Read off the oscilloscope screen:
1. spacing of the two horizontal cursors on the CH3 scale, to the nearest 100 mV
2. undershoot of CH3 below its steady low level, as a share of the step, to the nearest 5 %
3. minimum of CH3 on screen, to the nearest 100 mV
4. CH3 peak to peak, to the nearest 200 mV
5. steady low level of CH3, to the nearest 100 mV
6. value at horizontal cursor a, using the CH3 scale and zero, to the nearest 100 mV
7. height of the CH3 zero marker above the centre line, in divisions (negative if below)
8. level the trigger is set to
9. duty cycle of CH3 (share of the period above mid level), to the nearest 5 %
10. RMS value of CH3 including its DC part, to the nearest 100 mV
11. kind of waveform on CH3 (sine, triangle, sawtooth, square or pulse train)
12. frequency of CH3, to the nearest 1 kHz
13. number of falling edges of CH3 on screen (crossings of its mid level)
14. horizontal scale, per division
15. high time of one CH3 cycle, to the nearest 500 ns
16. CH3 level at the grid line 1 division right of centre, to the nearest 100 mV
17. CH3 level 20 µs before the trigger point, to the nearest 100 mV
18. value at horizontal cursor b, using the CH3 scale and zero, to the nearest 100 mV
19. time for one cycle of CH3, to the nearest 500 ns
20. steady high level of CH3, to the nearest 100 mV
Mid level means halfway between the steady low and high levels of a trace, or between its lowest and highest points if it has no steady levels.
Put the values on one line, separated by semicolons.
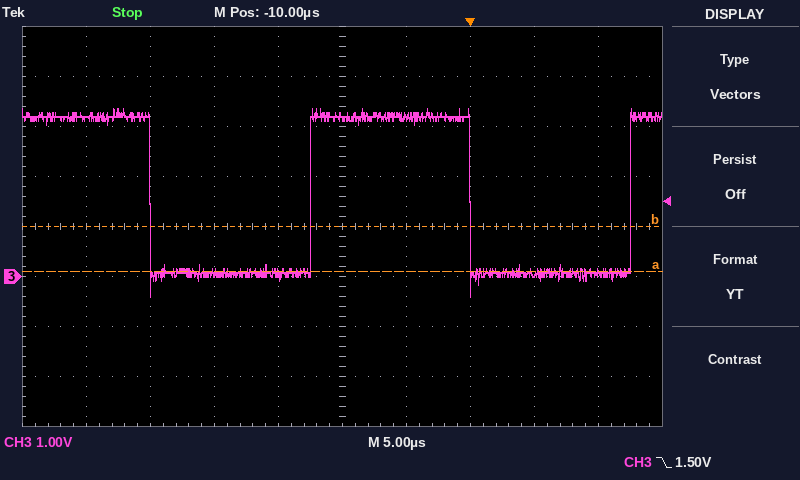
900 mV; 15 %; -400 mV; 3.8 V; 100 mV; 100 mV; -1.0 div; 1.50 V; 50 %; 2.3 V; square; 40 kHz; 2; 5 µs; 12.5 µs; 3.2 V; 100 mV; 1.0 V; 25.0 µs; 3.2 V
